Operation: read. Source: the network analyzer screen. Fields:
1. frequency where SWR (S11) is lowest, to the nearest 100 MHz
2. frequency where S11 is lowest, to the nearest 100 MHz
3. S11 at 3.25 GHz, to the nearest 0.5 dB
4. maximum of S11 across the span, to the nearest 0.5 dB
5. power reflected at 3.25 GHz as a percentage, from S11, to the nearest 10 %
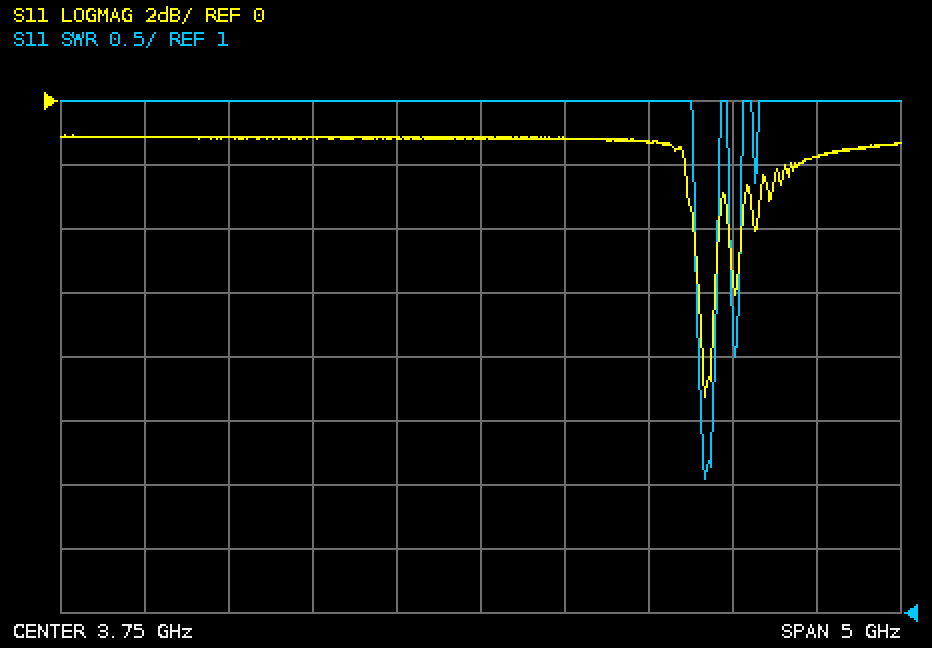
5.1 GHz
5.1 GHz
-1.0 dB
-1.0 dB
80 %
